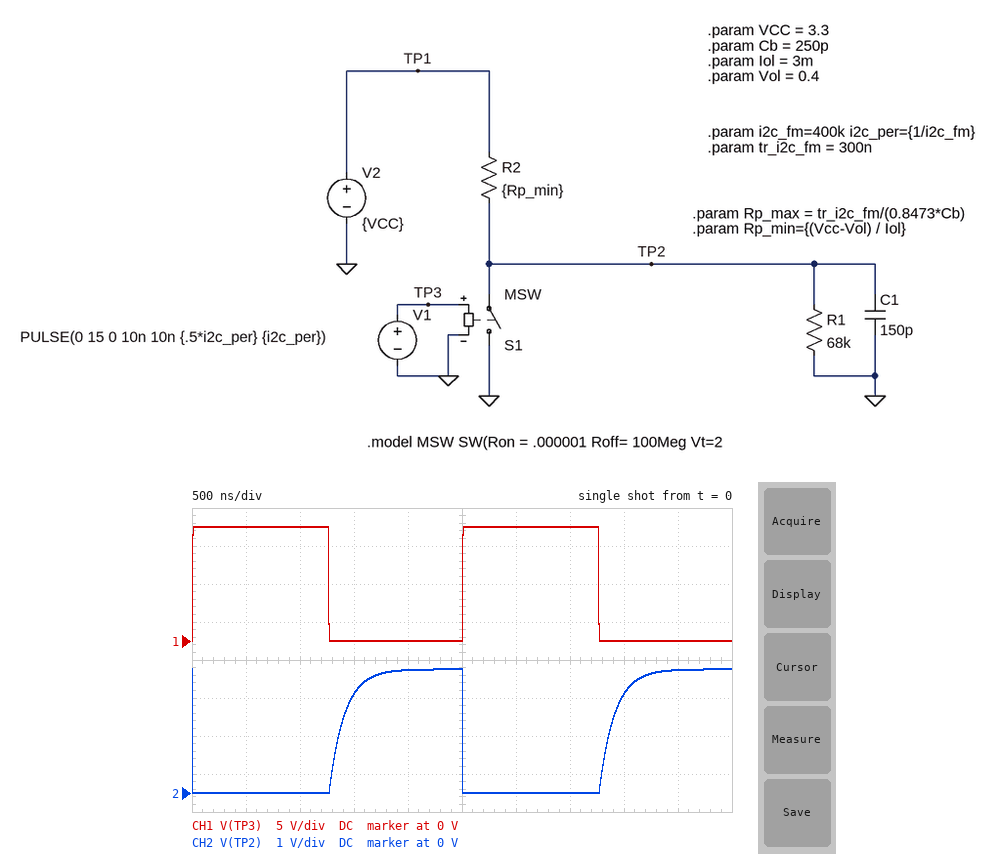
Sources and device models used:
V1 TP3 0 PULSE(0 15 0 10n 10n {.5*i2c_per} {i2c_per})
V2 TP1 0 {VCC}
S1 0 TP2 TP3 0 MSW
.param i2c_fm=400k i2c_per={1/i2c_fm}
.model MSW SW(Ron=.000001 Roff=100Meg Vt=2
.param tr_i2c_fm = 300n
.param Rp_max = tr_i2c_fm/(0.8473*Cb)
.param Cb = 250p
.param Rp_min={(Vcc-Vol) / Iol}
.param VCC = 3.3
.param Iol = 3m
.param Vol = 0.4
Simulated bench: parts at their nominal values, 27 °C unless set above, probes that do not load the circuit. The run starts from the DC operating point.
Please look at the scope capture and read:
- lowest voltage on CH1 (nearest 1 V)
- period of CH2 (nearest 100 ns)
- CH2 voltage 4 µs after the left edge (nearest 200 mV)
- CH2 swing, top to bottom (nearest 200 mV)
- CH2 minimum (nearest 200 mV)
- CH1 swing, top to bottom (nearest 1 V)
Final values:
0 V
2.5 µs
2.6 V
3.2 V
0 V
15 V
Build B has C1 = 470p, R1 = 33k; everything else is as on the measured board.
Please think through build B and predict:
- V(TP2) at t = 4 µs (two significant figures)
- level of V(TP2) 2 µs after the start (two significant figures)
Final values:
1.3 V
2.6 V
